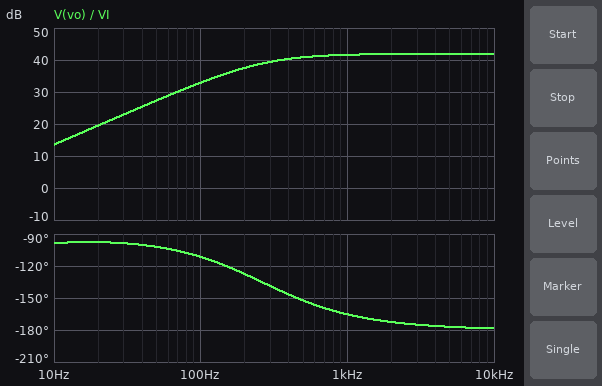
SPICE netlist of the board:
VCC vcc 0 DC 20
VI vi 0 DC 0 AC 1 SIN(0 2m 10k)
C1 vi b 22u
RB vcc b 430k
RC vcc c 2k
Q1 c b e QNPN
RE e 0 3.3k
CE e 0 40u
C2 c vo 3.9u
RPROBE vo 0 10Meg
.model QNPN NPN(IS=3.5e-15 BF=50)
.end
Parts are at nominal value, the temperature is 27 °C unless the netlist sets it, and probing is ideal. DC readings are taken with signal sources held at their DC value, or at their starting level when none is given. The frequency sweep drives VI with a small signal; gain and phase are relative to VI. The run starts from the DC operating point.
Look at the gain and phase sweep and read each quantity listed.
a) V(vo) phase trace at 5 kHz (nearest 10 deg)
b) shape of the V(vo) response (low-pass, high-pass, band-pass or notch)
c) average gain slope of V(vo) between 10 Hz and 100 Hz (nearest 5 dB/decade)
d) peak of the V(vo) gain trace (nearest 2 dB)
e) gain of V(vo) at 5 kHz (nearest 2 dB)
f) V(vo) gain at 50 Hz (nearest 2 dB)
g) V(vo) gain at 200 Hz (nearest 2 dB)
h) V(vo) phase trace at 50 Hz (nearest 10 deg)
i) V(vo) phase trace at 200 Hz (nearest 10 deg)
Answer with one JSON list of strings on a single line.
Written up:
["-180 deg", "high-pass", "20 dB/decade", "42 dB", "42 dB", "28 dB", "38 dB", "-100 deg", "-130 deg"]
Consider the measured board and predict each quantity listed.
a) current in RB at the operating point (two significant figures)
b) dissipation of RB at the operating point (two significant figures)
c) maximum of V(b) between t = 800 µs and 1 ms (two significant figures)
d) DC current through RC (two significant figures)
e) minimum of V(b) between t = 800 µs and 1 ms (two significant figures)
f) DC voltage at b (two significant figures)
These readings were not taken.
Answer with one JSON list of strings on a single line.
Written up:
["32 µA", "450 µW", "6.1 V", "1.6 mA", "6.1 V", "6.1 V"]
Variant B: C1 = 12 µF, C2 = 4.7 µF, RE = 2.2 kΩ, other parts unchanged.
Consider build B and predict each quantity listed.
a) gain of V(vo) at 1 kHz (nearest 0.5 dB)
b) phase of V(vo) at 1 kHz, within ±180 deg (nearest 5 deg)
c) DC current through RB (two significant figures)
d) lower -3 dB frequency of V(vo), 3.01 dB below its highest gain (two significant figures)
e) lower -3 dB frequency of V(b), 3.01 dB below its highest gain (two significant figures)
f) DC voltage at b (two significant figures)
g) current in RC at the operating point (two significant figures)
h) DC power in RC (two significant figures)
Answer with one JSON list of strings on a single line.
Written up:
["42.5 dB", "-165 deg", "36 µA", "300 Hz", "160 mHz", "4.7 V", "1.8 mA", "6.3 mW"]
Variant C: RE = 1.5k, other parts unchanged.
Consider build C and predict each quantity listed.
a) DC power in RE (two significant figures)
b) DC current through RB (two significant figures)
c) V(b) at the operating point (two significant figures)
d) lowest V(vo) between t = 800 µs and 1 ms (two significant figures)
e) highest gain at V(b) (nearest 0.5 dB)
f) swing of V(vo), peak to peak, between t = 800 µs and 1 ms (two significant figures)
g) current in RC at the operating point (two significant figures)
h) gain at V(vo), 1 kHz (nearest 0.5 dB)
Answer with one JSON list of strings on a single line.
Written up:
["5.7 mW", "38 µA", "3.6 V", "-300 mV", "0 dB", "590 mV", "1.9 mA", "43.0 dB"]
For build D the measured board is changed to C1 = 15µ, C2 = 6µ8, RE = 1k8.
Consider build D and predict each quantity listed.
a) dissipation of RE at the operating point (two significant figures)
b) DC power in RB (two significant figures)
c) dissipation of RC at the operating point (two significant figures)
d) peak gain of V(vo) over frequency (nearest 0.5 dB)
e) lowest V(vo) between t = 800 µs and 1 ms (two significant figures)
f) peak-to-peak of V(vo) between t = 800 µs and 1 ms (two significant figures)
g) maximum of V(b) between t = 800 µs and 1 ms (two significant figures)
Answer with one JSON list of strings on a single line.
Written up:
["6.4 mW", "590 µW", "6.8 mW", "43.0 dB", "-290 mV", "570 mV", "4.1 V"]
